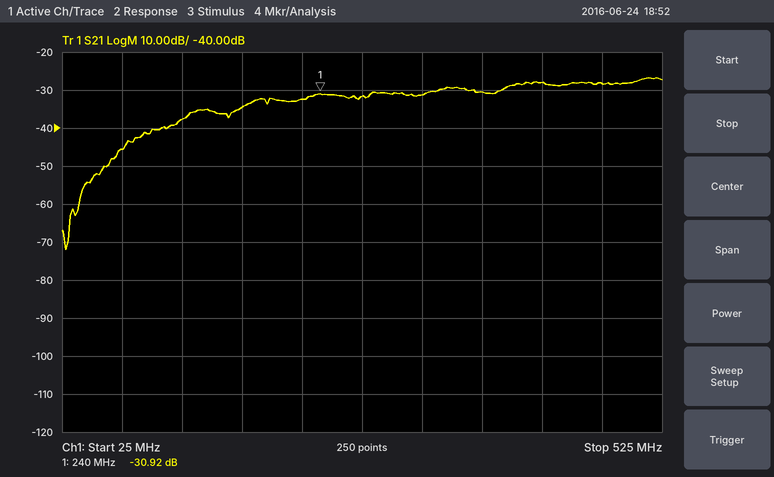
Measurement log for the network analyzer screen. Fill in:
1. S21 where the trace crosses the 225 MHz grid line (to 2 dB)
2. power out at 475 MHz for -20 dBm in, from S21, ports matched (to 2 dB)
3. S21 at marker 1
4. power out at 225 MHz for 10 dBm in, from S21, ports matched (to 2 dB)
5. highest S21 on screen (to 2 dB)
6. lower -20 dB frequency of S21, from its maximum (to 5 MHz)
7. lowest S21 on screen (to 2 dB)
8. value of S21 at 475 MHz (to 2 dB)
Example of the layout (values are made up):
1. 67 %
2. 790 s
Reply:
1. -32 dB
2. -48 dBm
3. -30.92 dB
4. -22 dBm
5. -26 dB
6. 70 MHz
7. -72 dB
8. -28 dB
